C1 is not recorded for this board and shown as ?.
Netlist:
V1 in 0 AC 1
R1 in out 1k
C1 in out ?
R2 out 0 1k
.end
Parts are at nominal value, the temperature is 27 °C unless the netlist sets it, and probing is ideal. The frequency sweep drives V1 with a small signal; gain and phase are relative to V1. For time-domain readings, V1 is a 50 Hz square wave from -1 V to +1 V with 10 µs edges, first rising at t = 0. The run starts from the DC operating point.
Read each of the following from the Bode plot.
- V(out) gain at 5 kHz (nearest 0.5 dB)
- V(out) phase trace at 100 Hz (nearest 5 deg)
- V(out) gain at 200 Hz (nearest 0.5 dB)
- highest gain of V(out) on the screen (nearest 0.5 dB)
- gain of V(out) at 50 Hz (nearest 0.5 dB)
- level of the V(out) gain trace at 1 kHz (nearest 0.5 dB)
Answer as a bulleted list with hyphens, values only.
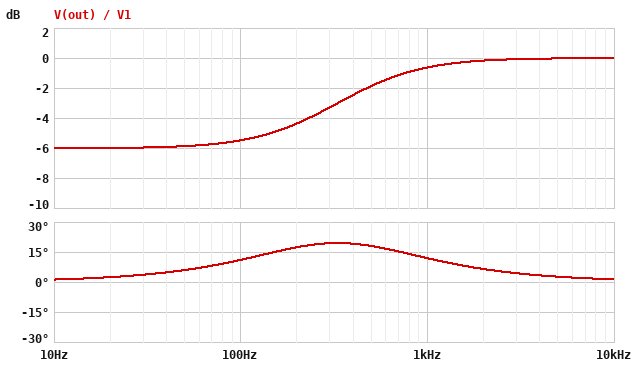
- 0 dB
- 10 deg
- -4.5 dB
- 0 dB
- -6.0 dB
- -0.5 dB
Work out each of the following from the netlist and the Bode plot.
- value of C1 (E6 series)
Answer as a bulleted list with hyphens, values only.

- 680 nF
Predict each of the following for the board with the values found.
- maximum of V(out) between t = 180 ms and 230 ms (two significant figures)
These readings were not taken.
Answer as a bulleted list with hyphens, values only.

- 1.5 V
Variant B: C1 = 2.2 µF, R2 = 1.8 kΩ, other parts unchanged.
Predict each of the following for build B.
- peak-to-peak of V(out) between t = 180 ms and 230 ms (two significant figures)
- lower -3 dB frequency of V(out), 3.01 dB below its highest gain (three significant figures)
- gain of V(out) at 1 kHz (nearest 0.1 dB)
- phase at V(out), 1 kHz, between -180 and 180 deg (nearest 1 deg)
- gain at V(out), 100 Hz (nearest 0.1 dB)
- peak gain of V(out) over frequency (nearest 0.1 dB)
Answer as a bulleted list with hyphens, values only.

- 2.7 V
- 46.9 Hz
- 0 dB
- 2 deg
- -1.7 dB
- 0 dB
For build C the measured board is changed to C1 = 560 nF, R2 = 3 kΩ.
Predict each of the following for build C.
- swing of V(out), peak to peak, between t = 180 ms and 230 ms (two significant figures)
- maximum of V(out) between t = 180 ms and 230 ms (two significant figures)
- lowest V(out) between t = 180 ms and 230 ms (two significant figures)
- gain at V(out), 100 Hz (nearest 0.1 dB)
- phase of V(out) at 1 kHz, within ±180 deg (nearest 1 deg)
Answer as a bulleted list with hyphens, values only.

- 2.5 V
- 1.2 V
- -1.2 V
- -2.3 dB
- 5 deg
